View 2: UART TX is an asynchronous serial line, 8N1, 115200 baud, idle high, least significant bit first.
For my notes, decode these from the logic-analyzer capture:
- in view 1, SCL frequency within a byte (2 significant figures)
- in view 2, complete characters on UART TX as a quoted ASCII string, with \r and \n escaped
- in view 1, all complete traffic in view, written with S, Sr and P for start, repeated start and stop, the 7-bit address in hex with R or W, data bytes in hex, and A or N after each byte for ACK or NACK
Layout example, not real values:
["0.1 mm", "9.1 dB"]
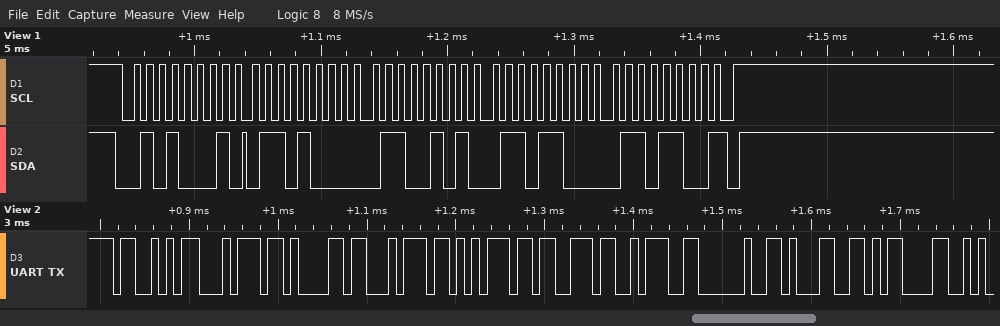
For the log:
["100 kHz", "\"Status: 1\\r\"", "S 28R A 68 A 65 A 6C A 6C N P"]
